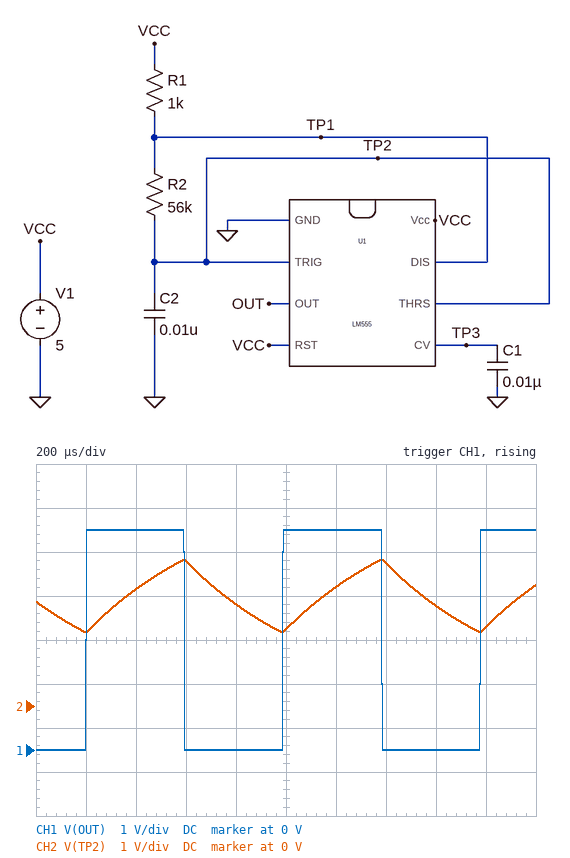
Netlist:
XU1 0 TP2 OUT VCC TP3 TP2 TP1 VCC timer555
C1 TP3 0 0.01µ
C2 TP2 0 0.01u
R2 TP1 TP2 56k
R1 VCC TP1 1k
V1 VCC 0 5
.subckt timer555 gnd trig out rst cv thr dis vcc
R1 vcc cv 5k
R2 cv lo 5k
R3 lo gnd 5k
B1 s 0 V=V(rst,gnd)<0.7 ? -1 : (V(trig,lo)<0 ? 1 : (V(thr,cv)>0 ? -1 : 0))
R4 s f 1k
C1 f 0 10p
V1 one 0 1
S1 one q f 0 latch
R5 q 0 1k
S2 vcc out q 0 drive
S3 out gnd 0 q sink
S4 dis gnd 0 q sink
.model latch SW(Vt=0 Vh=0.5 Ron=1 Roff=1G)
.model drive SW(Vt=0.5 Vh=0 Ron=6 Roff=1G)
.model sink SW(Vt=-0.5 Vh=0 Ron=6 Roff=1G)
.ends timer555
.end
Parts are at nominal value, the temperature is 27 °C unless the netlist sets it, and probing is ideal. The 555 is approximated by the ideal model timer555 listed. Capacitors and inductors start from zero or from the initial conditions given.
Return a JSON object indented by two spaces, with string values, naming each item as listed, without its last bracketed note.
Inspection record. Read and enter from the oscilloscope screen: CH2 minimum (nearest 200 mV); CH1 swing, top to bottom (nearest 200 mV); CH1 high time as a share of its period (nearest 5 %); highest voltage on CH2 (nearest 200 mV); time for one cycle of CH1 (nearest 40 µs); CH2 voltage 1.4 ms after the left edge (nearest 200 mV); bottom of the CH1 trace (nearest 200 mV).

{
  "CH2 minimum": "1.6 V",
  "CH1 swing, top to bottom": "5.0 V",
  "CH1 high time as a share of its period": "50 %",
  "highest voltage on CH2": "3.4 V",
  "time for one cycle of CH1": "800 µs",
  "CH2 voltage 1.4 ms after the left edge": "3.2 V",
  "bottom of the CH1 trace": "0 V"
}
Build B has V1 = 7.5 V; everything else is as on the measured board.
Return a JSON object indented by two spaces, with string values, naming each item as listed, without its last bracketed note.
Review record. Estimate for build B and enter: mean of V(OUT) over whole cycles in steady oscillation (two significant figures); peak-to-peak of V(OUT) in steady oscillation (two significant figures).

{
  "mean of V(OUT) over whole cycles in steady oscillation": "3.8 V",
  "peak-to-peak of V(OUT) in steady oscillation": "7.5 V"
}
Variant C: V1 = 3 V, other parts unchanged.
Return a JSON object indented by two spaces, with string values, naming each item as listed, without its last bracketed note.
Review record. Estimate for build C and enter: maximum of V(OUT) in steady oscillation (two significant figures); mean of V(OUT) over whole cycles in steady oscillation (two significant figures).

{
  "maximum of V(OUT) in steady oscillation": "3.0 V",
  "mean of V(OUT) over whole cycles in steady oscillation": "1.5 V"
}
